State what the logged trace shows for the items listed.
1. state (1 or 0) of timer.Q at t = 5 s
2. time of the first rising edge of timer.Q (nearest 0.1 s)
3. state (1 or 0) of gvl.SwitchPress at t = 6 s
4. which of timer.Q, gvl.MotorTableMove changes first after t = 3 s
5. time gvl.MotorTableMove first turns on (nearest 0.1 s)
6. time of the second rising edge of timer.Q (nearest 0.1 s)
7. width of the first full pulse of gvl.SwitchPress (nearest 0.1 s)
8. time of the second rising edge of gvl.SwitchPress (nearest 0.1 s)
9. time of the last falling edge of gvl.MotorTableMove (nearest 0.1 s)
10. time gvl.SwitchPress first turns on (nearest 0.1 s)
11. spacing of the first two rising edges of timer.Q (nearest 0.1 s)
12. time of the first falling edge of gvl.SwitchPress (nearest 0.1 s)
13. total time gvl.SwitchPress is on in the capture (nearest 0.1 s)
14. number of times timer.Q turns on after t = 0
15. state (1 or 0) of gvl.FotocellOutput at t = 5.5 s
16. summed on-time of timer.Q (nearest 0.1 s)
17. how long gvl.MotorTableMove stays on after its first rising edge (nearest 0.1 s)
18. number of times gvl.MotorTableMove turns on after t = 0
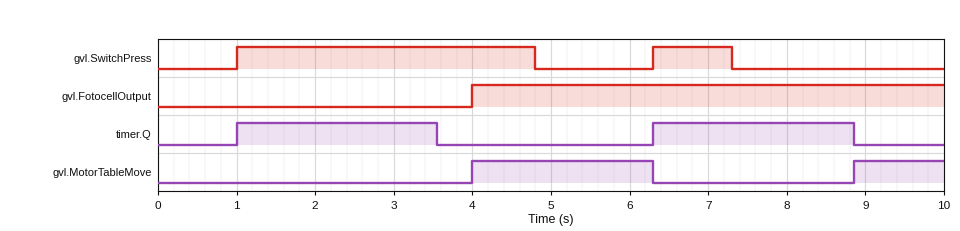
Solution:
0
1.0 s
0
timer.Q
4.0 s
6.3 s
3.8 s
6.3 s
6.3 s
1.0 s
5.3 s
4.8 s
4.8 s
2
1
5.1 s
2.3 s
2
